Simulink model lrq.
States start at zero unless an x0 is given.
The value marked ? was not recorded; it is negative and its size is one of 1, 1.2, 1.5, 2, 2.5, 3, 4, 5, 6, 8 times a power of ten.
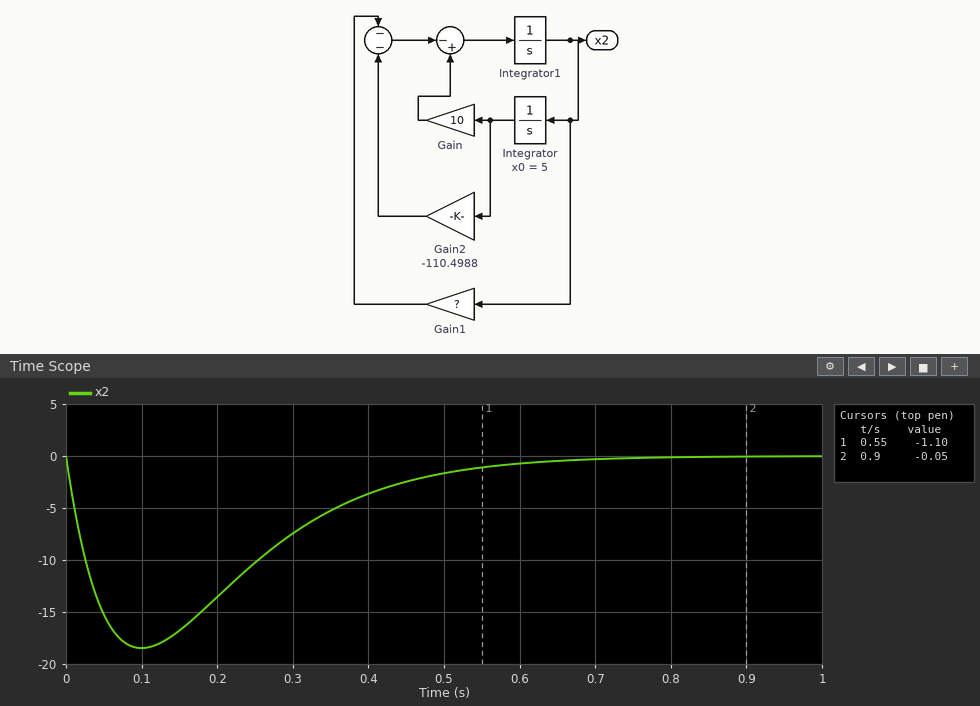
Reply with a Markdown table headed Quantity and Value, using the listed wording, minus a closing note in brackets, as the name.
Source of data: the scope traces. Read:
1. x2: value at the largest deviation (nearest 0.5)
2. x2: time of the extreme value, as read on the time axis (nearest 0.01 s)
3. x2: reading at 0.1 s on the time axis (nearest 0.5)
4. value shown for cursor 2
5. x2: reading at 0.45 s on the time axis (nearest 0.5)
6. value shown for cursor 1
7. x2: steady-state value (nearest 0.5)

| Quantity | Value |
|---|---|
| x2: value at the largest deviation | -18.5 |
| x2: time of the extreme value, as read on the time axis | 0.10 s |
| x2: reading at 0.1 s on the time axis | -18.5 |
| value shown for cursor 2 | -0.05 |
| x2: reading at 0.45 s on the time axis | -2.5 |
| value shown for cursor 1 | -1.10 |
| x2: steady-state value | 0.0 |
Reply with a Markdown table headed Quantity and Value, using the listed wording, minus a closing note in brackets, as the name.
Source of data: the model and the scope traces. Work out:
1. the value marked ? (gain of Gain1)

| Quantity | Value |
|---|---|
| the value marked ? | -20 |
